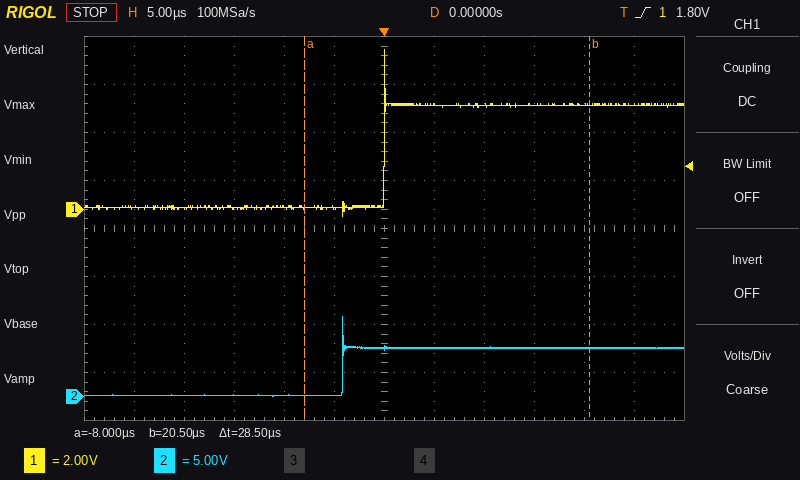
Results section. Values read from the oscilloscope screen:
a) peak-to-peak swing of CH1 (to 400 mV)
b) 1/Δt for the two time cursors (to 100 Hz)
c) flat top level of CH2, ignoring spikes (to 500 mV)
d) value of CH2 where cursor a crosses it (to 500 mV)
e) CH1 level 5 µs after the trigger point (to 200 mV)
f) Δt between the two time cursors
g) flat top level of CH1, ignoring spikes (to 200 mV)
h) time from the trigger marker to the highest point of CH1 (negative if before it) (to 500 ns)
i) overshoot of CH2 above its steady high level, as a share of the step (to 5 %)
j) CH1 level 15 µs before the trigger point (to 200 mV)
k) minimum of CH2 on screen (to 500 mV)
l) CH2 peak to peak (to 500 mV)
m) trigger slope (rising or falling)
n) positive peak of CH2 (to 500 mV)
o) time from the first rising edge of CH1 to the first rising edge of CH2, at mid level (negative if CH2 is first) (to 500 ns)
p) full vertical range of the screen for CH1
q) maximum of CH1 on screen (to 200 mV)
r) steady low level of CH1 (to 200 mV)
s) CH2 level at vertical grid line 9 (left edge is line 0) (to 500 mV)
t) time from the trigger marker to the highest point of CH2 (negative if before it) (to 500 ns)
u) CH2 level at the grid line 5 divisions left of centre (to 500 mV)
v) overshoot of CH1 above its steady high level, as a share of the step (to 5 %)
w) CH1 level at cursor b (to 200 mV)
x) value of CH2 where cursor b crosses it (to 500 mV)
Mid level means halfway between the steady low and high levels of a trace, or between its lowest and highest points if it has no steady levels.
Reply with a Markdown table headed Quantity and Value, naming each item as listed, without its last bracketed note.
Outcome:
| Quantity | Value |
|---|---|
| peak-to-peak swing of CH1 | 6.8 V |
| 1/Δt for the two time cursors | 35.1 kHz |
| flat top level of CH2, ignoring spikes | 5.0 V |
| value of CH2 where cursor a crosses it | 0.0 V |
| CH1 level 5 µs after the trigger point | 4.4 V |
| Δt between the two time cursors | 28.5 µs |
| flat top level of CH1, ignoring spikes | 4.4 V |
| time from the trigger marker to the highest point of CH1 (negative if before it) | 0.0 µs |
| overshoot of CH2 above its steady high level, as a share of the step | 65 % |
| CH1 level 15 µs before the trigger point | 0.0 V |
| minimum of CH2 on screen | 0.0 V |
| CH2 peak to peak | 8.5 V |
| trigger slope | rising |
| positive peak of CH2 | 8.5 V |
| time from the first rising edge of CH1 to the first rising edge of CH2, at mid level (negative if CH2 is first) | -4.0 µs |
| full vertical range of the screen for CH1 | 16 V |
| maximum of CH1 on screen | 6.6 V |
| steady low level of CH1 | 0.0 V |
| CH2 level at vertical grid line 9 (left edge is line 0) | 5.0 V |
| time from the trigger marker to the highest point of CH2 (negative if before it) | -4.0 µs |
| CH2 level at the grid line 5 divisions left of centre | 0.0 V |
| overshoot of CH1 above its steady high level, as a share of the step | 55 % |
| CH1 level at cursor b | 4.4 V |
| value of CH2 where cursor b crosses it | 5.0 V |
